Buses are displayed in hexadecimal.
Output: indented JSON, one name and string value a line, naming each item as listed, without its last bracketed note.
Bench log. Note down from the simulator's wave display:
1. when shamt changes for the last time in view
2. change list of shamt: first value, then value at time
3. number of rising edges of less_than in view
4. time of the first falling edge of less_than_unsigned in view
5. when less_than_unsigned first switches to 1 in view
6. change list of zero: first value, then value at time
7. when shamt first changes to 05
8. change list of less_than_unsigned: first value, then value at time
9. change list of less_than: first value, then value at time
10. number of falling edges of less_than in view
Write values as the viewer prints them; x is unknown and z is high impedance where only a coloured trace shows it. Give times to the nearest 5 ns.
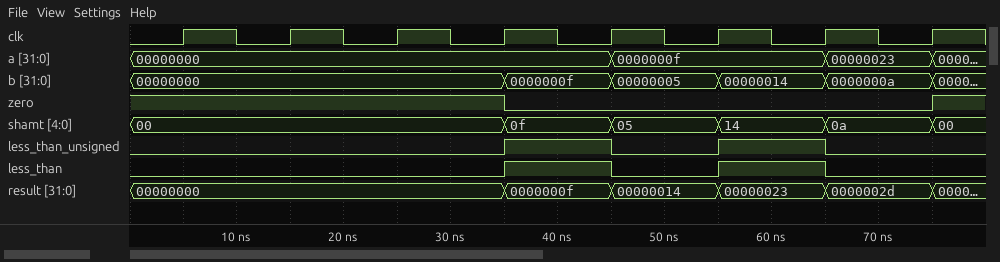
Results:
{
  "when shamt changes for the last time in view": "75 ns",
  "change list of shamt: first value, then value at time": "00, 0f at 35 ns, 05 at 45 ns, 14 at 55 ns, 0a at 65 ns, 00 at 75 ns",
  "number of rising edges of less_than in view": "2",
  "time of the first falling edge of less_than_unsigned in view": "45 ns",
  "when less_than_unsigned first switches to 1 in view": "35 ns",
  "change list of zero: first value, then value at time": "1, 0 at 35 ns, 1 at 75 ns",
  "when shamt first changes to 05": "45 ns",
  "change list of less_than_unsigned: first value, then value at time": "0, 1 at 35 ns, 0 at 45 ns, 1 at 55 ns, 0 at 65 ns",
  "change list of less_than: first value, then value at time": "0, 1 at 35 ns, 0 at 45 ns, 1 at 55 ns, 0 at 65 ns",
  "number of falling edges of less_than in view": "2"
}
